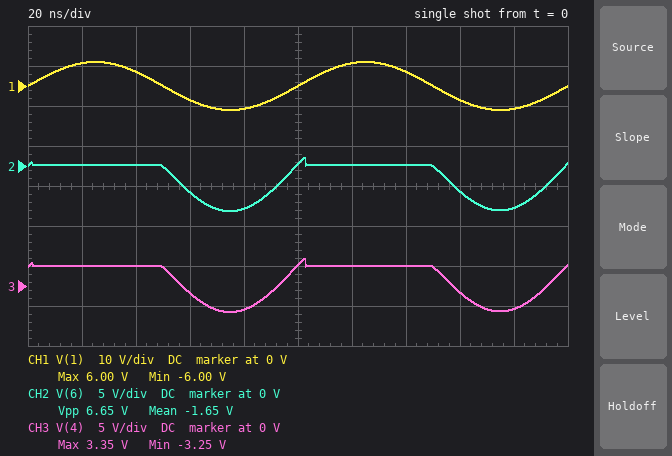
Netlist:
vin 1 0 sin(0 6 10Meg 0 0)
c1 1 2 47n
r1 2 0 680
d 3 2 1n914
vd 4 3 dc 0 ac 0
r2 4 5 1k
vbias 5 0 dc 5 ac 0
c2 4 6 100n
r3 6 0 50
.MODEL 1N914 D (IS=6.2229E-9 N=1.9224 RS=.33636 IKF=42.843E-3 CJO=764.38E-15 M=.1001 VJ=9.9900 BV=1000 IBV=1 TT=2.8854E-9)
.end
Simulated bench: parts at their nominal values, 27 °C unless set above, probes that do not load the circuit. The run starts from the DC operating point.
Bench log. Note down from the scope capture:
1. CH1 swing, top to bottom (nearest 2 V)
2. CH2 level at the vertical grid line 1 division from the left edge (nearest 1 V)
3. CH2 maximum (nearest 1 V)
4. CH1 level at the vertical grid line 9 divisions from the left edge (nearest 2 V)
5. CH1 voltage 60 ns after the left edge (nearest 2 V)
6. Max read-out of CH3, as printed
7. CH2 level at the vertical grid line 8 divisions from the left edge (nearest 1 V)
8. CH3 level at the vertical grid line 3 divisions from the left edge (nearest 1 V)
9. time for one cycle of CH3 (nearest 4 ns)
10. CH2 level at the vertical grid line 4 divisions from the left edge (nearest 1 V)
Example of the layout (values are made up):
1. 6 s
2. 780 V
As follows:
1. 12 V
2. 0 V
3. 1 V
4. -6 V
5. -4 V
6. 3.35 V
7. -3 V
8. -1 V
9. 100 ns
10. -5 V
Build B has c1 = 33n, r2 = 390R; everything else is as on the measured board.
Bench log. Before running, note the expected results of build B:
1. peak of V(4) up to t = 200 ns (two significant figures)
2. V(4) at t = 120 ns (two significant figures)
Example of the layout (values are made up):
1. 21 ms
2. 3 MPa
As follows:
1. 4.4 V
2. 3.6 V
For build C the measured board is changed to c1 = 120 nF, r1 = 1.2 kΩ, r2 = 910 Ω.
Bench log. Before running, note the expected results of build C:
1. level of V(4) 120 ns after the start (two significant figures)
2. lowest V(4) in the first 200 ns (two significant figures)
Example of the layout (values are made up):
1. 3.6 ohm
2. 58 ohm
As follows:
1. 3.2 V
2. -2.6 V
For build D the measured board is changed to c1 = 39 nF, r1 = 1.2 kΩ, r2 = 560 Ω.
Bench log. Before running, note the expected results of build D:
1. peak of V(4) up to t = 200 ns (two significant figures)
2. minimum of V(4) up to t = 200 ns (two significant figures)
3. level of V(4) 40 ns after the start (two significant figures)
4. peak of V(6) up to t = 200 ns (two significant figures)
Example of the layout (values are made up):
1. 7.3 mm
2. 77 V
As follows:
1. 4.6 V
2. -2.0 V
3. 3.7 V
4. 980 mV
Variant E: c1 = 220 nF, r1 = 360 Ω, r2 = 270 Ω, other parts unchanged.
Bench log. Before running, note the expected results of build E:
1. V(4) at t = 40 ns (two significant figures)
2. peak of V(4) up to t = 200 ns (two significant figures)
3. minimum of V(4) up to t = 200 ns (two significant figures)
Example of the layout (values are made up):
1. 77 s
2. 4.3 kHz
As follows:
1. 3.4 V
2. 4.3 V
3. -2.6 V
